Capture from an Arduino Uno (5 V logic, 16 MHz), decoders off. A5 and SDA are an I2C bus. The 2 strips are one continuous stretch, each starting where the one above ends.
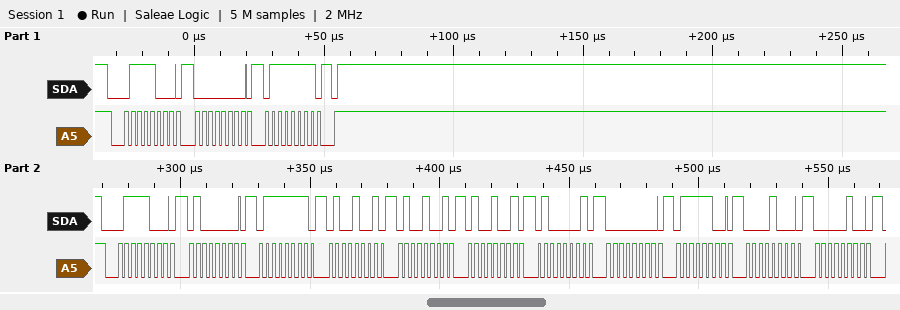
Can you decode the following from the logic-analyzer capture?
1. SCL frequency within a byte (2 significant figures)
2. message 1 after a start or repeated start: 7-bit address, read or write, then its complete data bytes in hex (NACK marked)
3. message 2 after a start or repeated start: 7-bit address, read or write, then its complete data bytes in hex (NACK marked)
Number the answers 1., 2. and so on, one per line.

1. 400 kHz
2. 0x3C write: 00 7F
3. 0x3C write: 40 7F 49 49 49 41 00 7C 08 04
